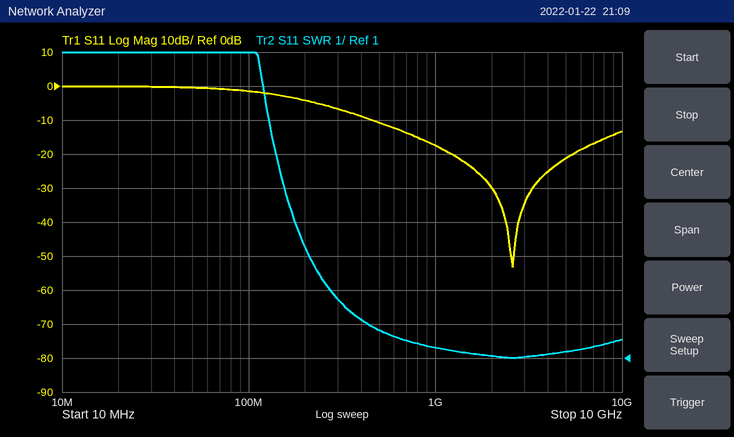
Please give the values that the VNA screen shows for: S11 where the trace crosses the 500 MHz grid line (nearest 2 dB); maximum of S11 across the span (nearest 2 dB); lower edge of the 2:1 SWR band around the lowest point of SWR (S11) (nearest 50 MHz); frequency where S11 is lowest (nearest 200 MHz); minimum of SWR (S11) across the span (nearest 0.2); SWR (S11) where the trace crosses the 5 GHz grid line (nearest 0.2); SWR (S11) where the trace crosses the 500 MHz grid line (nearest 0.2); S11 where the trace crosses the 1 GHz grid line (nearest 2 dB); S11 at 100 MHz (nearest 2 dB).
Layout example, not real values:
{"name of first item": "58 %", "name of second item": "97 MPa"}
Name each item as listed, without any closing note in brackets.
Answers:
{"S11 where the trace crosses the 500 MHz grid line": "-10 dB", "maximum of S11 across the span": "0 dB", "lower edge of the 2:1 SWR band around the lowest point of SWR (S11)": "450 MHz", "frequency where S11 is lowest": "2.6 GHz", "minimum of SWR (S11) across the span": "1.0", "SWR (S11) where the trace crosses the 5 GHz grid line": "1.2", "SWR (S11) where the trace crosses the 500 MHz grid line": "1.8", "S11 where the trace crosses the 1 GHz grid line": "-18 dB", "S11 at 100 MHz": "-2 dB"}
